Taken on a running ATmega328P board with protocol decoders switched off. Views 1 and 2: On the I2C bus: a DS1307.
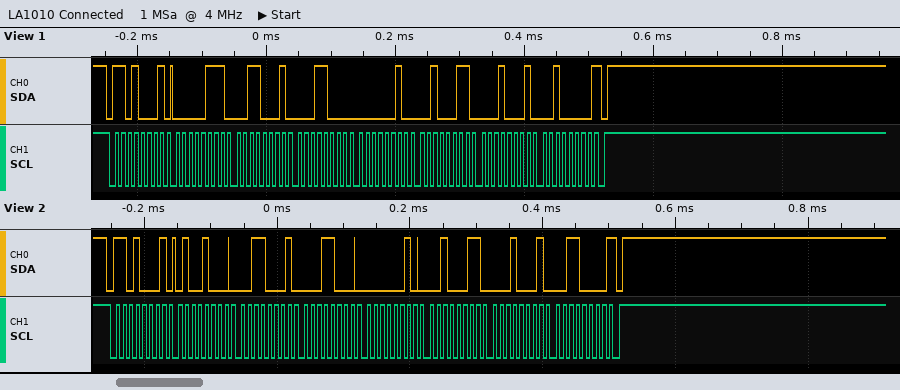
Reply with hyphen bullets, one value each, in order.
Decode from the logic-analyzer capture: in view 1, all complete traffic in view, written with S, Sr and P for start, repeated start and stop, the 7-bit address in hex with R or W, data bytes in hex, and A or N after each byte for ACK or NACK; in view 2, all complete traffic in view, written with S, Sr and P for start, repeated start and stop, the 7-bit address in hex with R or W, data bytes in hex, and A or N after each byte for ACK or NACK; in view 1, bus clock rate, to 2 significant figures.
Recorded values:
- S 68R A 07 A 31 A 18 A 02 A 23 A 11 A 20 N P
- S 68R A 48 A 31 A 18 A 02 A 23 A 11 A 30 N P
- 100 kHz
